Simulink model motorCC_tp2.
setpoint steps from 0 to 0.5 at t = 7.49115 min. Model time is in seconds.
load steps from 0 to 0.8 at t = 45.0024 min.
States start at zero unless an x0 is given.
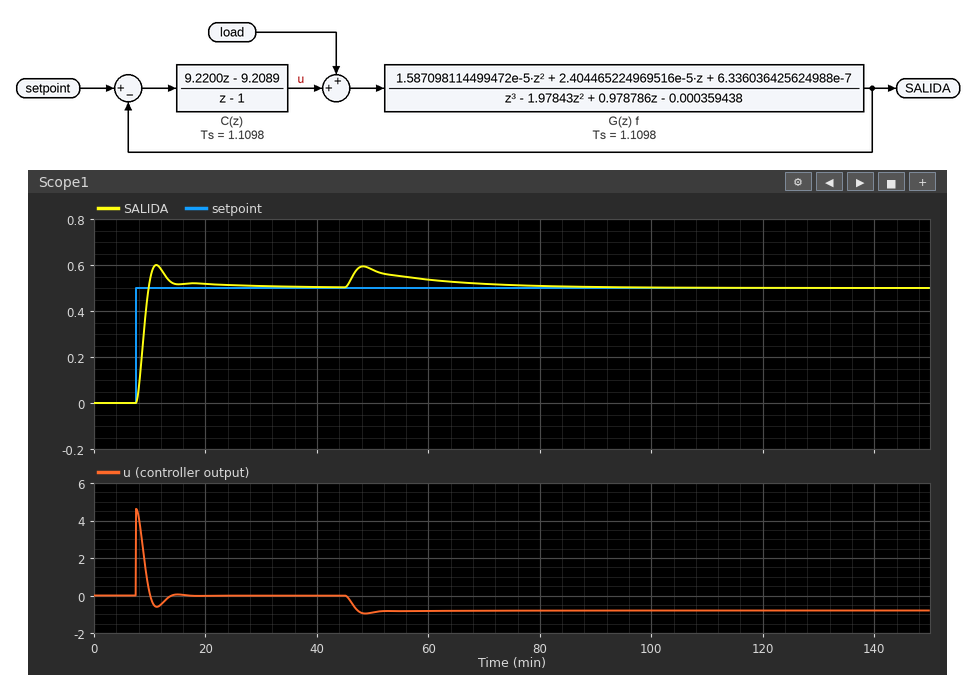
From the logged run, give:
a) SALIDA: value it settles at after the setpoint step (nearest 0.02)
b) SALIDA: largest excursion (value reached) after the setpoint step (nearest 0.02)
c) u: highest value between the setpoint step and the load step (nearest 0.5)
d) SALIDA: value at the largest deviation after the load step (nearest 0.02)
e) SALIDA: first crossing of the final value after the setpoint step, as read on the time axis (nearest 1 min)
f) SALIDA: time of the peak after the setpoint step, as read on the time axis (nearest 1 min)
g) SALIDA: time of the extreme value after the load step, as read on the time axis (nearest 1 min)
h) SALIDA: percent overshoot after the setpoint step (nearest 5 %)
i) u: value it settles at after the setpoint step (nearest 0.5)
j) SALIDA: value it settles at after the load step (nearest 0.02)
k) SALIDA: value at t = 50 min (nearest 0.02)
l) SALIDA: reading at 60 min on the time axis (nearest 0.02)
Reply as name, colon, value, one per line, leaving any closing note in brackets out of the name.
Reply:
SALIDA: value it settles at after the setpoint step: 0.50
SALIDA: largest excursion (value reached) after the setpoint step: 0.60
u: highest value between the setpoint step and the load step: 4.5
SALIDA: value at the largest deviation after the load step: 0.60
SALIDA: first crossing of the final value after the setpoint step, as read on the time axis: 10 min
SALIDA: time of the peak after the setpoint step, as read on the time axis: 11 min
SALIDA: time of the extreme value after the load step, as read on the time axis: 48 min
SALIDA: percent overshoot after the setpoint step: 20 %
u: value it settles at after the setpoint step: 0.0
SALIDA: value it settles at after the load step: 0.50
SALIDA: value at t = 50 min: 0.58
SALIDA: reading at 60 min on the time axis: 0.54
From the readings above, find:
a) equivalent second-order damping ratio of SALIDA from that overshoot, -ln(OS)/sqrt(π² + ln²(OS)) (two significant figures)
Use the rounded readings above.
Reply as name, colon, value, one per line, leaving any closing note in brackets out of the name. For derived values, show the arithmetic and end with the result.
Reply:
equivalent second-order damping ratio of SALIDA from that overshoot, -ln(OS)/sqrt(π² + ln²(OS)): ln(0.2) = -1.609; 1.609 / sqrt(9.870 + 2.590) = 0.46
